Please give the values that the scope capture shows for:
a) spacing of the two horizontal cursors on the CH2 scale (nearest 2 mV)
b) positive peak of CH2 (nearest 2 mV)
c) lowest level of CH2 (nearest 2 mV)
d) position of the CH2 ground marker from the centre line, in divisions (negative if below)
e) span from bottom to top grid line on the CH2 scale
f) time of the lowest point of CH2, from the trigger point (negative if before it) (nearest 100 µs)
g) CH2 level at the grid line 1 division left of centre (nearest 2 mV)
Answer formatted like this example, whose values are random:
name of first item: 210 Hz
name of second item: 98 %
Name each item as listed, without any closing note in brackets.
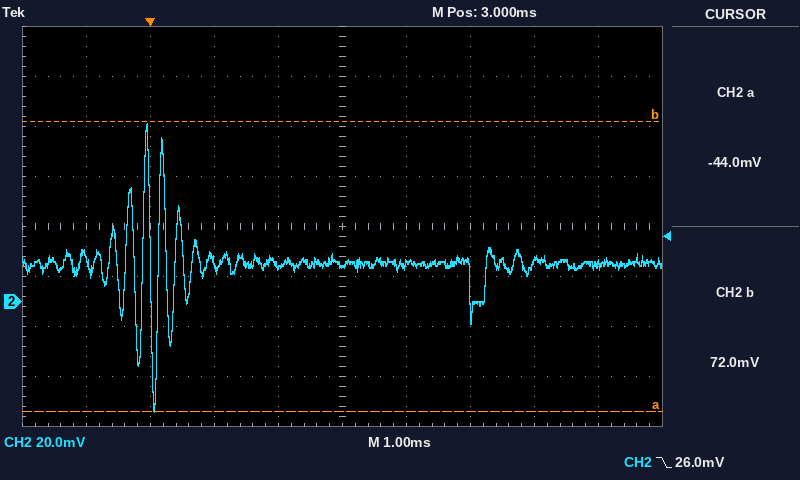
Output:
spacing of the two horizontal cursors on the CH2 scale: 116 mV
positive peak of CH2: 72 mV
lowest level of CH2: -44 mV
position of the CH2 ground marker from the centre line, in divisions: -1.5 div
span from bottom to top grid line on the CH2 scale: 160 mV
time of the lowest point of CH2, from the trigger point (negative if before it): +100 µs
CH2 level at the grid line 1 division left of centre: 14 mV
